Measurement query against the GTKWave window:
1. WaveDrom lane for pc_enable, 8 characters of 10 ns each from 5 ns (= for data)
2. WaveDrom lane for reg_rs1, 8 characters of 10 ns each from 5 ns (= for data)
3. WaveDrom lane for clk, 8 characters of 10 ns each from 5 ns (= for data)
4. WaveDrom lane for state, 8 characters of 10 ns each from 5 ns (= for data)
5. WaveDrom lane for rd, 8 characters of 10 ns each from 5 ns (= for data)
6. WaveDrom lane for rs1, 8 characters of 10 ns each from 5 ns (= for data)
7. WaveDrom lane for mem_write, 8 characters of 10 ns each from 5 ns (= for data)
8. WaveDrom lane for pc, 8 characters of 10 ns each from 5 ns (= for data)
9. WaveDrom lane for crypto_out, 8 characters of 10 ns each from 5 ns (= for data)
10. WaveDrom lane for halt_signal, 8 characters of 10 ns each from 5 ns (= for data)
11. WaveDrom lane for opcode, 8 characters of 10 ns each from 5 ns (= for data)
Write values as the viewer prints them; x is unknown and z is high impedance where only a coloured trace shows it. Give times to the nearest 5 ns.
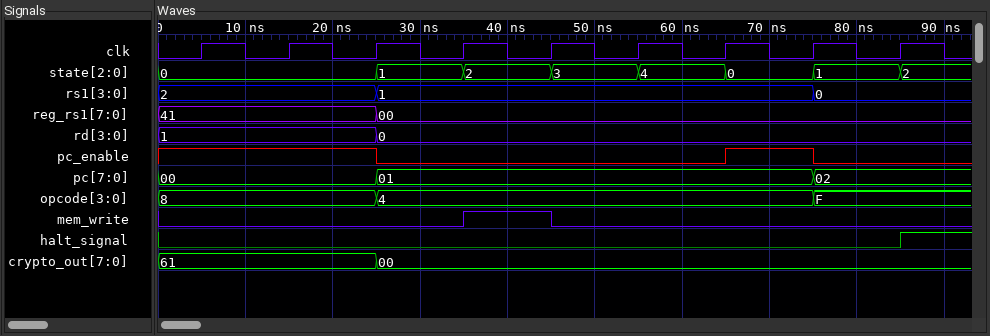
{name: 'pc_enable', wave: '1.0...10'}
{name: 'reg_rs1', wave: '=.=.....', data: '41 00'}
{name: 'clk', wave: 'p.......'}
{name: 'state', wave: '=.======', data: '0 1 2 3 4 0 1'}
{name: 'rd', wave: '=.=.....', data: '1 0'}
{name: 'rs1', wave: '=.=....=', data: '2 1 0'}
{name: 'mem_write', wave: '0..10...'}
{name: 'pc', wave: '=.=....=', data: '00 01 02'}
{name: 'crypto_out', wave: '=.=.....', data: '61 00'}
{name: 'halt_signal', wave: '0.......'}
{name: 'opcode', wave: '=.=....=', data: '8 4 F'}
